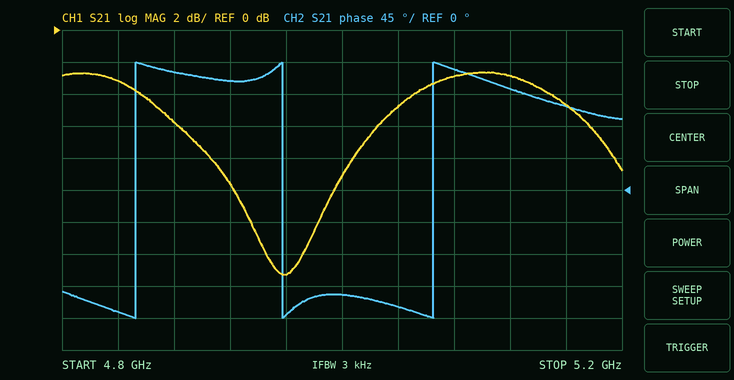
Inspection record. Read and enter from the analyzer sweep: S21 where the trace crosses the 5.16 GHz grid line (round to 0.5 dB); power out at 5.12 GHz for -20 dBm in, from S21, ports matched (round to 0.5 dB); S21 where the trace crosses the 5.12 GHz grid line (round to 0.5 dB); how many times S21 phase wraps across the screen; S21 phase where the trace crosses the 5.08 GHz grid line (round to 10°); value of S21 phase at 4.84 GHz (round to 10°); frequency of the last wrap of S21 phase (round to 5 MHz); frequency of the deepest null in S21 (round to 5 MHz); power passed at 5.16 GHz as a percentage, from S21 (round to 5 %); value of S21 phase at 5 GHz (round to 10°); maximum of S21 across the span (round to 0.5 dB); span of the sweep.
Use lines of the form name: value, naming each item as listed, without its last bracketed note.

S21 where the trace crosses the 5.16 GHz grid line: -4.5 dB
power out at 5.12 GHz for -20 dBm in, from S21, ports matched: -23.0 dBm
S21 where the trace crosses the 5.12 GHz grid line: -3.0 dB
how many times S21 phase wraps across the screen: 3
S21 phase where the trace crosses the 5.08 GHz grid line: 170°
value of S21 phase at 4.84 GHz: -170°
frequency of the last wrap of S21 phase: 5.065 GHz
frequency of the deepest null in S21: 4.960 GHz
power passed at 5.16 GHz as a percentage, from S21: 35 %
value of S21 phase at 5 GHz: -150°
maximum of S21 across the span: -2.5 dB
span of the sweep: 400 MHz
